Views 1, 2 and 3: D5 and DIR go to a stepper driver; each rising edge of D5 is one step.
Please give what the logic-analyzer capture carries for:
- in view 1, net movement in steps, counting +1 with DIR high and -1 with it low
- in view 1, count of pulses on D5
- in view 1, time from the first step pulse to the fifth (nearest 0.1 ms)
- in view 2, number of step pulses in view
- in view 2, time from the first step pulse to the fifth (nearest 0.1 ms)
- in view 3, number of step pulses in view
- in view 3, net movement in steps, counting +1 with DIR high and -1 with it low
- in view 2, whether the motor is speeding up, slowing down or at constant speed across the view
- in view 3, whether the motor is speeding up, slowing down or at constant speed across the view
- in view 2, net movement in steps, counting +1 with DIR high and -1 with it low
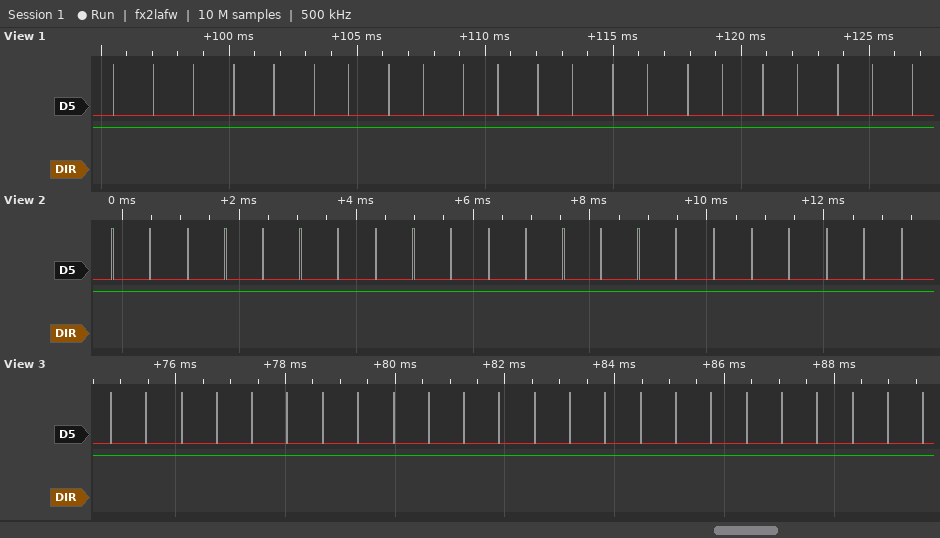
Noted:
+22
22
6.3 ms
22
2.6 ms
24
+24
constant speed
constant speed
+22
